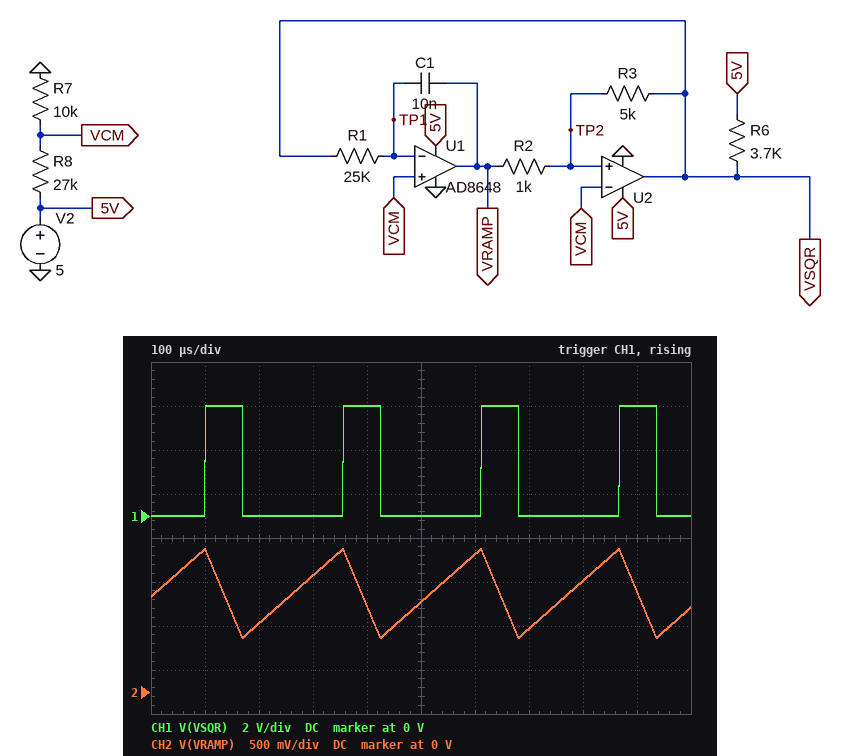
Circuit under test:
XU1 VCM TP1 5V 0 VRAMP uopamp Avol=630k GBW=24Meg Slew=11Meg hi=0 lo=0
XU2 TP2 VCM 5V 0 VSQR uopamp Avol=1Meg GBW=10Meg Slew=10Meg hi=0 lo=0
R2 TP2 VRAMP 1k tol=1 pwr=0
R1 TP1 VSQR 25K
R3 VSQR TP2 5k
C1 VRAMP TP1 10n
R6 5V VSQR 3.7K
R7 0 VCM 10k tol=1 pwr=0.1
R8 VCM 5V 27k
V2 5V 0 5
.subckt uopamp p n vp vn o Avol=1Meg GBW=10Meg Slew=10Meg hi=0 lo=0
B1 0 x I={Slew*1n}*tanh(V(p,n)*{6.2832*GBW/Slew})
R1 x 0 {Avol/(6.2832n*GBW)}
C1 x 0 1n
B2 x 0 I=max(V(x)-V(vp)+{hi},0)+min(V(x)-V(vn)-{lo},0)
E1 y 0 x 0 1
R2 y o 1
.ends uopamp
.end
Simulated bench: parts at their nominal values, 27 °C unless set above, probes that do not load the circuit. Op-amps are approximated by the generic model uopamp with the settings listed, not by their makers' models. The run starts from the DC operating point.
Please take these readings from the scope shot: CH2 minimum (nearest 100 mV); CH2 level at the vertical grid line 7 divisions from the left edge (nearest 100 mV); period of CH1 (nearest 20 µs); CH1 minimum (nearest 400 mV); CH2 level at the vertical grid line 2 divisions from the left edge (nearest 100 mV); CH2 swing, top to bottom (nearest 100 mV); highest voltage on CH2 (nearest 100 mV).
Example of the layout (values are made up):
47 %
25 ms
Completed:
600 mV
700 mV
260 µs
0 V
800 mV
1.0 V
1.6 V
